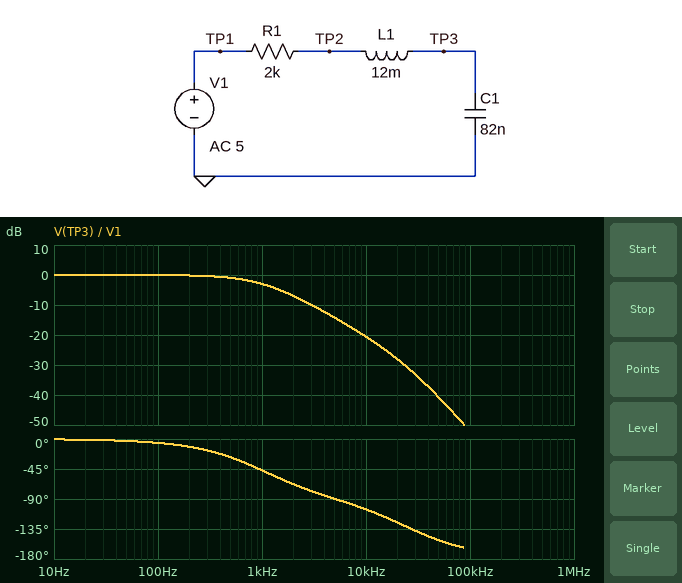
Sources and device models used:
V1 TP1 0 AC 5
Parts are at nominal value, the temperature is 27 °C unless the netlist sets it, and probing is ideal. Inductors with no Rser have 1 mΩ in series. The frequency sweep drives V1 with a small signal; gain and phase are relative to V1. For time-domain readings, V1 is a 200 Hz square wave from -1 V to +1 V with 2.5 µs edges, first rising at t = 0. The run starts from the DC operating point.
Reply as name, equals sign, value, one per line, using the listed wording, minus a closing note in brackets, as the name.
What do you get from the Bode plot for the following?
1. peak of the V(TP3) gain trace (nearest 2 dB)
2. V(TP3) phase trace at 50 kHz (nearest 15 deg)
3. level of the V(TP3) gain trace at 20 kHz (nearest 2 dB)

peak of the V(TP3) gain trace = 0 dB
V(TP3) phase trace at 50 kHz = -150 deg
level of the V(TP3) gain trace at 20 kHz = -28 dB
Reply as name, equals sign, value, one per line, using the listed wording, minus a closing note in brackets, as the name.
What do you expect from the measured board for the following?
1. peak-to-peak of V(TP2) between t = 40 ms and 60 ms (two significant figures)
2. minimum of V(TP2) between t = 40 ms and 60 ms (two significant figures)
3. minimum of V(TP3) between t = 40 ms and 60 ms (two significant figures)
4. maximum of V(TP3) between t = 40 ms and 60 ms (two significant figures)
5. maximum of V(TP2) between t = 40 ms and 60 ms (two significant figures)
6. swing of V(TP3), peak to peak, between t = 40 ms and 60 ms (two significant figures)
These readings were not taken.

peak-to-peak of V(TP2) between t = 40 ms and 60 ms = 2.0 V
minimum of V(TP2) between t = 40 ms and 60 ms = -1.0 V
minimum of V(TP3) between t = 40 ms and 60 ms = -1.0 V
maximum of V(TP3) between t = 40 ms and 60 ms = 1.0 V
maximum of V(TP2) between t = 40 ms and 60 ms = 1.0 V
swing of V(TP3), peak to peak, between t = 40 ms and 60 ms = 2.0 V
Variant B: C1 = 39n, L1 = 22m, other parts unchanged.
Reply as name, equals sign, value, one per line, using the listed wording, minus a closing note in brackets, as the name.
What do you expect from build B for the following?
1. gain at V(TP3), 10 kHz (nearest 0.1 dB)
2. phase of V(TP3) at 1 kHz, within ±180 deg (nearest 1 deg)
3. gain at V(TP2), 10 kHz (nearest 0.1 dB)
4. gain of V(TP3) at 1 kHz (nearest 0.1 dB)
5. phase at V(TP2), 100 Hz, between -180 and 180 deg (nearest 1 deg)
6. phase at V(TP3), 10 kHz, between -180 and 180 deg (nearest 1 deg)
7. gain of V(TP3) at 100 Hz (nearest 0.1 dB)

gain at V(TP3), 10 kHz = -14.7 dB
phase of V(TP3) at 1 kHz, within ±180 deg = -27 deg
gain at V(TP2), 10 kHz = -7.2 dB
gain of V(TP3) at 1 kHz = -0.7 dB
phase at V(TP2), 100 Hz, between -180 and 180 deg = -3 deg
phase at V(TP3), 10 kHz, between -180 and 180 deg = -116 deg
gain of V(TP3) at 100 Hz = 0 dB
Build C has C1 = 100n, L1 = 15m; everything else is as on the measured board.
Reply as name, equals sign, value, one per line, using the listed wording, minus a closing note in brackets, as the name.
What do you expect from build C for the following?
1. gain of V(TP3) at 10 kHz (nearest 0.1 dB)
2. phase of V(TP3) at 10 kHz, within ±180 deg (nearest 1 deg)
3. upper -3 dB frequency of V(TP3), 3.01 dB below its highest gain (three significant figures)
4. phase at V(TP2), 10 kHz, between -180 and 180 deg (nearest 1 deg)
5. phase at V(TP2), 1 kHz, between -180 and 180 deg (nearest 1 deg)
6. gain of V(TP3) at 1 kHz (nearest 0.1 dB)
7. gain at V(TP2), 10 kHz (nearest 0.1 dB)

gain of V(TP3) at 10 kHz = -22.6 dB
phase of V(TP3) at 10 kHz, within ±180 deg = -111 deg
upper -3 dB frequency of V(TP3), 3.01 dB below its highest gain = 827 Hz
phase at V(TP2), 10 kHz, between -180 and 180 deg = 69 deg
phase at V(TP2), 1 kHz, between -180 and 180 deg = -53 deg
gain of V(TP3) at 1 kHz = -3.9 dB
gain at V(TP2), 10 kHz = -8.8 dB
